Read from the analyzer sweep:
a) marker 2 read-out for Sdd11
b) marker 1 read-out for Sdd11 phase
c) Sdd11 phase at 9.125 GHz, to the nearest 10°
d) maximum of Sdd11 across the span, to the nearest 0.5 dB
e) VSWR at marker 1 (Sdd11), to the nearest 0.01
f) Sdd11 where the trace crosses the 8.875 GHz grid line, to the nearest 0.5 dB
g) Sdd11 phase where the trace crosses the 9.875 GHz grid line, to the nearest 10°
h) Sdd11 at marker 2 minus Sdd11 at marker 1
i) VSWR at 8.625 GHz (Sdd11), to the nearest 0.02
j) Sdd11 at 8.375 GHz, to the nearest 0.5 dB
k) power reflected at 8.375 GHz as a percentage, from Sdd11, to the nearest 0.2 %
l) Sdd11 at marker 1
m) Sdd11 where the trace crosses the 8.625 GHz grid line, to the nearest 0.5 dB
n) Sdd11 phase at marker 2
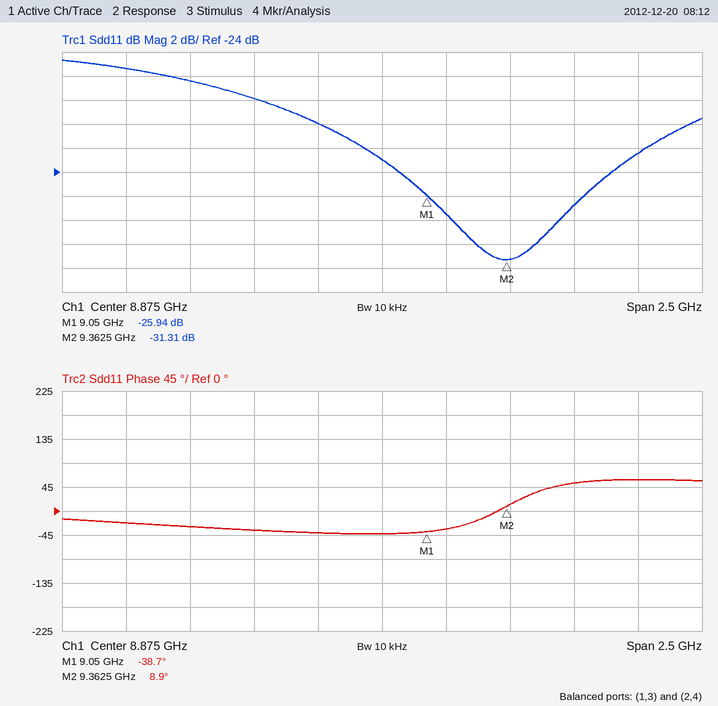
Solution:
-31.31 dB
-38.7°
-30°
-14.5 dB
1.11
-23.0 dB
60°
-5.37 dB
1.22
-18.0 dB
1.6 %
-25.94 dB
-20.0 dB
8.9°
